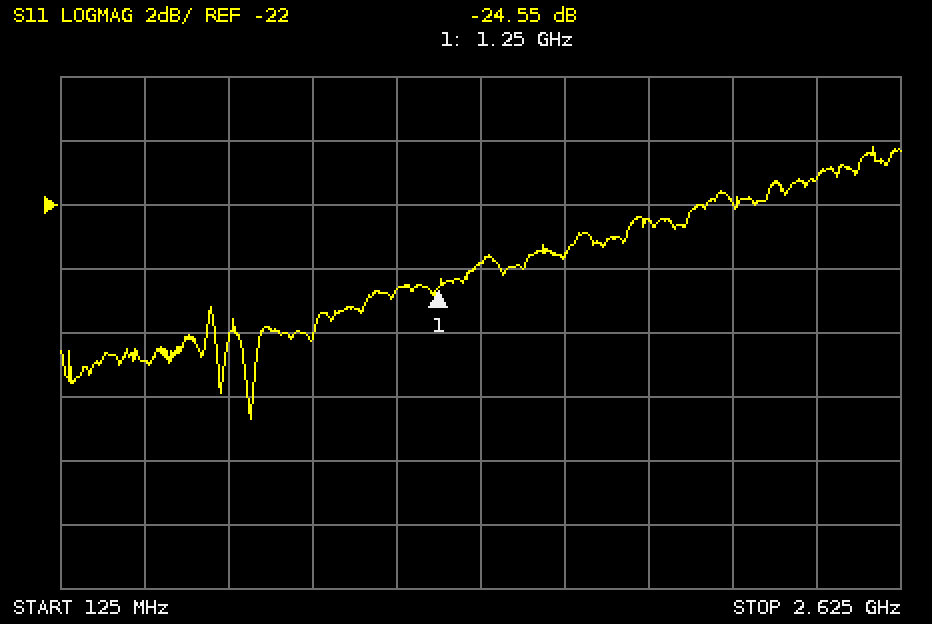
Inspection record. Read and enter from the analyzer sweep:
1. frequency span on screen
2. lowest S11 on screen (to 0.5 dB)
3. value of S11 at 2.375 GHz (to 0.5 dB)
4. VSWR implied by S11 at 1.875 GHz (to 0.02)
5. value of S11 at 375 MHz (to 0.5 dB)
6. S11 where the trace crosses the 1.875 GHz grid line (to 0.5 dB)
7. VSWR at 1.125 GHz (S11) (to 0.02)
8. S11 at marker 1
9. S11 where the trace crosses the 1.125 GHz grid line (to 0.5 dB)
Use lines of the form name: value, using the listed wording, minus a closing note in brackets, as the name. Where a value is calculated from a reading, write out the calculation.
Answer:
frequency span on screen: 2.5 GHz
lowest S11 on screen: -28.5 dB
value of S11 at 2.375 GHz: -21.0 dB
VSWR implied by S11 at 1.875 GHz: |Γ| = 10^(-22.5/20) = 0.0750; VSWR = (1 + 0.0750)/(1 − 0.0750) ≈ 1.16
value of S11 at 375 MHz: -27.0 dB
S11 where the trace crosses the 1.875 GHz grid line: -22.5 dB
VSWR at 1.125 GHz (S11): |Γ| = 10^(-24.5/20) = 0.0596; VSWR = (1 + 0.0596)/(1 − 0.0596) ≈ 1.13, so 1.12 to the nearest 0.02
S11 at marker 1: -24.55 dB
S11 where the trace crosses the 1.125 GHz grid line: -24.5 dB
